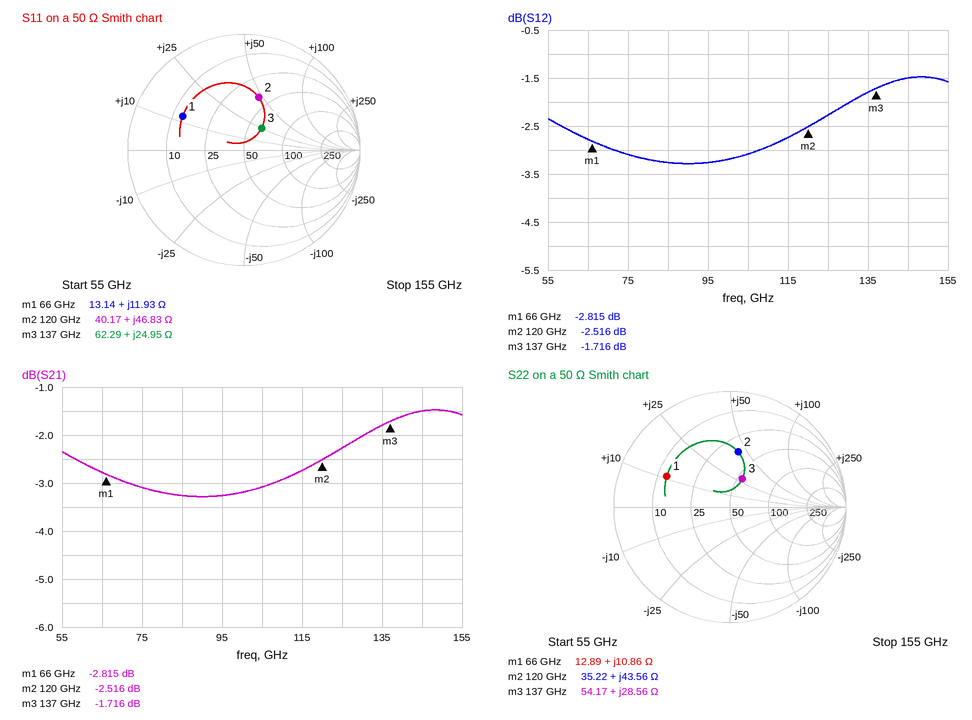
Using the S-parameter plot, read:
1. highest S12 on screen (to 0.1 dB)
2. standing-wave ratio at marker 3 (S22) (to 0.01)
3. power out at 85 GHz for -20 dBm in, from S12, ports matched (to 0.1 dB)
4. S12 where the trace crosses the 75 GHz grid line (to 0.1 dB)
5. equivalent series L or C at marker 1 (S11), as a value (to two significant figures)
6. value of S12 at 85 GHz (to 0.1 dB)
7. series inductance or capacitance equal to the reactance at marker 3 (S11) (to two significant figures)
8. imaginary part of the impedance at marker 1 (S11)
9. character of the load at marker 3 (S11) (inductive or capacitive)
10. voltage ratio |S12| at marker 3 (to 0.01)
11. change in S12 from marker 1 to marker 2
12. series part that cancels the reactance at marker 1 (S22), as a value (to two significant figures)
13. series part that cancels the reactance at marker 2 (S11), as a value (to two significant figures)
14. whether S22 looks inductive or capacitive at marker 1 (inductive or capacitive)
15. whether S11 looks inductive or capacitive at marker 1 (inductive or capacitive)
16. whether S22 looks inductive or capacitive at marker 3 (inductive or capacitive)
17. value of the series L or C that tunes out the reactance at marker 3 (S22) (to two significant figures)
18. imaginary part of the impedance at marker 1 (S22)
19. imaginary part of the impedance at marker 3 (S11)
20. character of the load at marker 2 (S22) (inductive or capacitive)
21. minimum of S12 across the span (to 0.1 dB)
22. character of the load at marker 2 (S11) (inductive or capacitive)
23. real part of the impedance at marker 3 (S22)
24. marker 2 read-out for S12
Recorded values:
-1.5 dB
1.73
-23.3 dBm
-3.1 dB
29 pH
-3.3 dB
29 pH
+11.93 Ω
inductive
0.82
0.299 dB
220 fF
28 fF
inductive
inductive
inductive
41 fF
+10.86 Ω
+24.95 Ω
inductive
-3.3 dB
inductive
54.17 Ω
-2.516 dB
